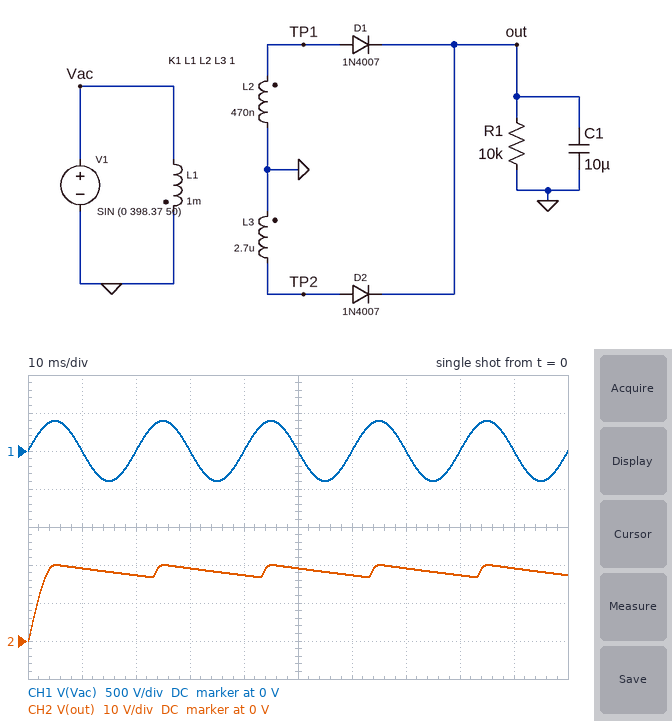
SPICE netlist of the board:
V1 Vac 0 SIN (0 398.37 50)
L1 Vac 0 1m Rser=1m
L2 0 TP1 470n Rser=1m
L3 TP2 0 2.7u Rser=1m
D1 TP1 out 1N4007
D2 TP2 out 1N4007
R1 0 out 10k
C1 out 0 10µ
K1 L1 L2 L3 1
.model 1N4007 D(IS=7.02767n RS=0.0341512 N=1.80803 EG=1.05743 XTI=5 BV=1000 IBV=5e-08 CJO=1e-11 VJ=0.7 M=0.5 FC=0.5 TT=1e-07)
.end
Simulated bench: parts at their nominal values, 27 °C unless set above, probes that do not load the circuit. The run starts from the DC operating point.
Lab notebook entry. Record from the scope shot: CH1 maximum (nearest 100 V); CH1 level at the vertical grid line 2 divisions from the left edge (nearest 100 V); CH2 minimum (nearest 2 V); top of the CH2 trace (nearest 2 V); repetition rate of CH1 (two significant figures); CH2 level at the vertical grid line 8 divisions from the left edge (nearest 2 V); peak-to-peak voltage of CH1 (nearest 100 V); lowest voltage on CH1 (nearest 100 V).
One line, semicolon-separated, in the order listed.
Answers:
400 V; 0 V; 0 V; 20 V; 50 Hz; 18 V; 800 V; -400 V
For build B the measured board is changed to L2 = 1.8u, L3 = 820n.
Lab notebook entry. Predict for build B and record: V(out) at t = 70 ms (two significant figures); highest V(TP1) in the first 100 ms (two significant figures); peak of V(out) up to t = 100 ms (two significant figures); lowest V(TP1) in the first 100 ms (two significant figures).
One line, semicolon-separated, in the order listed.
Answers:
14 V; 17 V; 16 V; -17 V
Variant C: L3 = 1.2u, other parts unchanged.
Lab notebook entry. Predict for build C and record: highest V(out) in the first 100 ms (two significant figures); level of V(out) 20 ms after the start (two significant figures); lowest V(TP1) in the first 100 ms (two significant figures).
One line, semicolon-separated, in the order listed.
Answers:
13 V; 11 V; -8.6 V
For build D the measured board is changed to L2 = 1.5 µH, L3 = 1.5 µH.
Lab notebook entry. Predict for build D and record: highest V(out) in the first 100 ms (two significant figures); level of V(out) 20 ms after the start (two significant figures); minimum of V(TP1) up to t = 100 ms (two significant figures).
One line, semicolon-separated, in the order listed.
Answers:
15 V; 14 V; -15 V
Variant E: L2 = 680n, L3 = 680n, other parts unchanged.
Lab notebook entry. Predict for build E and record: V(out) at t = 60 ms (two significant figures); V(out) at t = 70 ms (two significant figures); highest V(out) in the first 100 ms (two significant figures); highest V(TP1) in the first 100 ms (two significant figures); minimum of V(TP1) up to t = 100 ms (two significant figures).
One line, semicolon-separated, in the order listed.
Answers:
9.4 V; 9.3 V; 9.8 V; 10 V; -10 V
